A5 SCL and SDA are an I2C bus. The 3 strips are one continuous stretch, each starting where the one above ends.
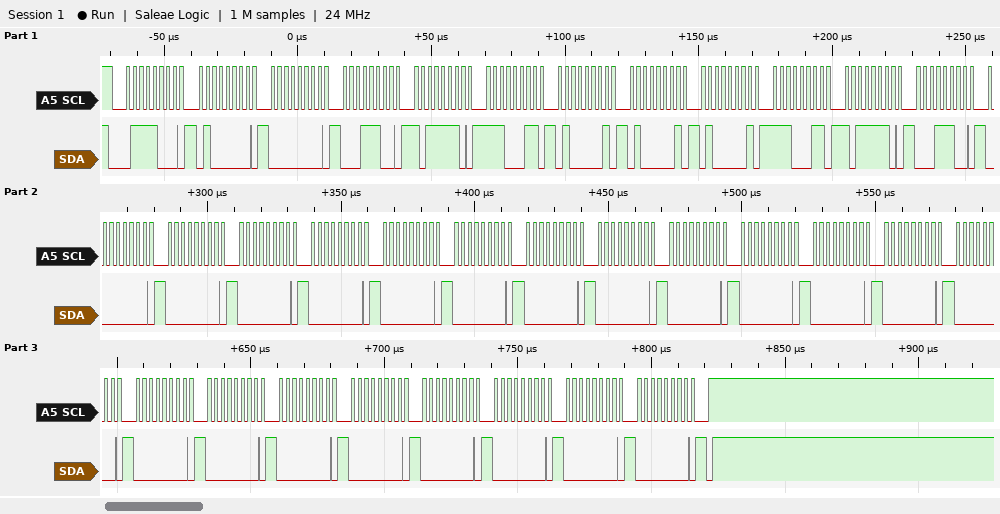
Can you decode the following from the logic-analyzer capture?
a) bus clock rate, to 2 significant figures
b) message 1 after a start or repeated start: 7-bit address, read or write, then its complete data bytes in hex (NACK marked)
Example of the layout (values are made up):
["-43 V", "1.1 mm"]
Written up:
["400 kHz", "0x3C write: 40 00 1C BE E3 41 41 41 E3 BE 1C 00 00 00 00 00 00 00 00 00 00 00 00 00 00 00 00 00 00 00 00 00"]
